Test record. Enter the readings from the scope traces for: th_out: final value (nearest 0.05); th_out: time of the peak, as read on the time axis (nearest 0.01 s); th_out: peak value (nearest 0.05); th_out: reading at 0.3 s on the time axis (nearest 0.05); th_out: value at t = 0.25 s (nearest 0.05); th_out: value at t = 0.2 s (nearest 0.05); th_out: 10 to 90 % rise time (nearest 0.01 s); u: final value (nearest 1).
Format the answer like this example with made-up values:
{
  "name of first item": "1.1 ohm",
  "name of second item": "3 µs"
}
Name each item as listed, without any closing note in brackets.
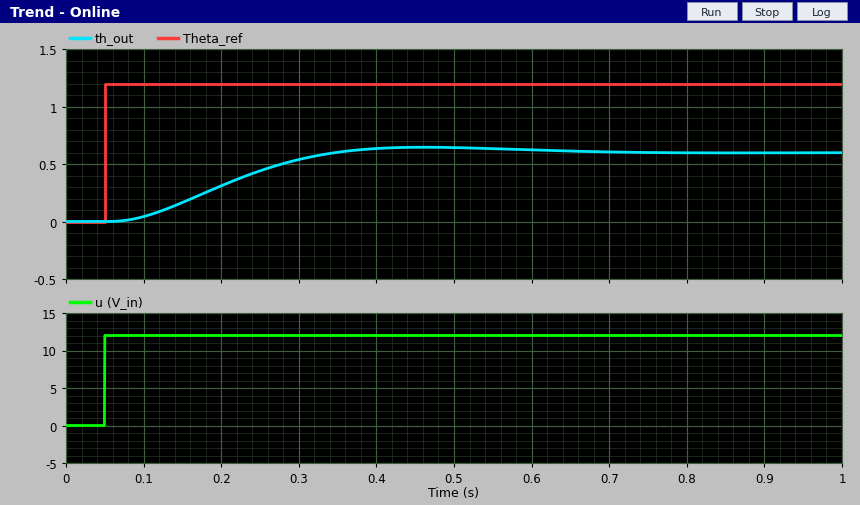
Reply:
{
  "th_out: final value": "0.60",
  "th_out: time of the peak, as read on the time axis": "0.46 s",
  "th_out: peak value": "0.65",
  "th_out: reading at 0.3 s on the time axis": "0.55",
  "th_out: value at t = 0.25 s": "0.45",
  "th_out: value at t = 0.2 s": "0.30",
  "th_out: 10 to 90 % rise time": "0.19 s",
  "u: final value": "12"
}
